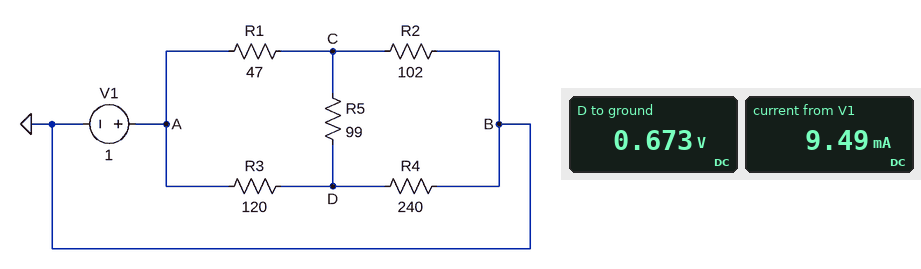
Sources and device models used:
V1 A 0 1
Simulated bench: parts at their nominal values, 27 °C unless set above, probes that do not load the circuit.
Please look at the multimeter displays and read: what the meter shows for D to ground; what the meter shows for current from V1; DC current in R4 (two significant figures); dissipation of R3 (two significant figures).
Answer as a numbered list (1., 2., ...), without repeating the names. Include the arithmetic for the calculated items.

1. 0.673 V
2. 9.49 mA
3. (673 mV) / 240 Ω = 2.8 mA
4. (1 V - 673 mV)^2 / 120 Ω = 890 µW
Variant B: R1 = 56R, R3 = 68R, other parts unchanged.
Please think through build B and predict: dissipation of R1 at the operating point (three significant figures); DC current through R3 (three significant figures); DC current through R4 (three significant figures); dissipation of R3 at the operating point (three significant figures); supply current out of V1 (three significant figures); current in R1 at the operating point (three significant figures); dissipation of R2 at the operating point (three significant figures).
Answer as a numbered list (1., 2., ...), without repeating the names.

1. 1.93 mW
2. 3.80 mA
3. 3.09 mA
4. 982 µW
5. 9.67 mA
6. 5.87 mA
7. 4.42 mW
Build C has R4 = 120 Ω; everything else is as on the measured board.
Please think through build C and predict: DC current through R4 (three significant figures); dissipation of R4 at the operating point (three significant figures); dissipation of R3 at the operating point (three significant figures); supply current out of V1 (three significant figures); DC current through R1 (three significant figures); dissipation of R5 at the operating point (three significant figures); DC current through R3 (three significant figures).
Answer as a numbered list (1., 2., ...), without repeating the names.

1. 4.65 mA
2. 2.59 mW
3. 1.63 mW
4. 11.1 mA
5. 7.37 mA
6. 92.3 µW
7. 3.68 mA
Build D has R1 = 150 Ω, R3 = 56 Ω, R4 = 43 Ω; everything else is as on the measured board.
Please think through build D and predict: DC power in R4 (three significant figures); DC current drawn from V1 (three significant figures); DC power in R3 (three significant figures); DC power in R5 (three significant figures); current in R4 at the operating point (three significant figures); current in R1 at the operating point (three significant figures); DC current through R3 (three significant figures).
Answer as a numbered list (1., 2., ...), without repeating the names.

1. 4.31 mW
2. 14.1 mA
3. 5.79 mW
4. 2.56 µW
5. 10.0 mA
6. 3.90 mA
7. 10.2 mA
